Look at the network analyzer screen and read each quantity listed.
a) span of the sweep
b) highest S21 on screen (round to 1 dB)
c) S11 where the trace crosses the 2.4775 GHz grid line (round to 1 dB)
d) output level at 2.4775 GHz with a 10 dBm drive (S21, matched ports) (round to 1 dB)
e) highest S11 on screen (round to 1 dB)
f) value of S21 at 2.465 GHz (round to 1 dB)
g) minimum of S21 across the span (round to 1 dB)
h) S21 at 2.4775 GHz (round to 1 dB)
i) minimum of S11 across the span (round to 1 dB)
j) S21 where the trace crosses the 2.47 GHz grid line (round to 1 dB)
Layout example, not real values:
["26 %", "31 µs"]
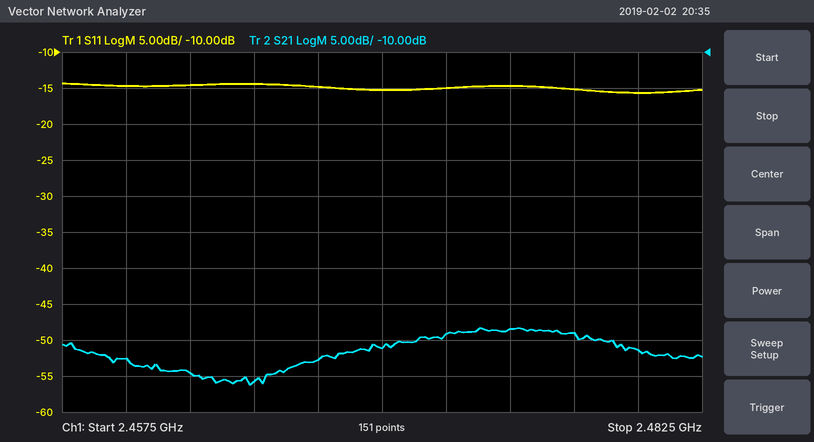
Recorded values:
["25 MHz", "-48 dB", "-15 dB", "-39 dBm", "-14 dB", "-56 dB", "-56 dB", "-49 dB", "-16 dB", "-51 dB"]
